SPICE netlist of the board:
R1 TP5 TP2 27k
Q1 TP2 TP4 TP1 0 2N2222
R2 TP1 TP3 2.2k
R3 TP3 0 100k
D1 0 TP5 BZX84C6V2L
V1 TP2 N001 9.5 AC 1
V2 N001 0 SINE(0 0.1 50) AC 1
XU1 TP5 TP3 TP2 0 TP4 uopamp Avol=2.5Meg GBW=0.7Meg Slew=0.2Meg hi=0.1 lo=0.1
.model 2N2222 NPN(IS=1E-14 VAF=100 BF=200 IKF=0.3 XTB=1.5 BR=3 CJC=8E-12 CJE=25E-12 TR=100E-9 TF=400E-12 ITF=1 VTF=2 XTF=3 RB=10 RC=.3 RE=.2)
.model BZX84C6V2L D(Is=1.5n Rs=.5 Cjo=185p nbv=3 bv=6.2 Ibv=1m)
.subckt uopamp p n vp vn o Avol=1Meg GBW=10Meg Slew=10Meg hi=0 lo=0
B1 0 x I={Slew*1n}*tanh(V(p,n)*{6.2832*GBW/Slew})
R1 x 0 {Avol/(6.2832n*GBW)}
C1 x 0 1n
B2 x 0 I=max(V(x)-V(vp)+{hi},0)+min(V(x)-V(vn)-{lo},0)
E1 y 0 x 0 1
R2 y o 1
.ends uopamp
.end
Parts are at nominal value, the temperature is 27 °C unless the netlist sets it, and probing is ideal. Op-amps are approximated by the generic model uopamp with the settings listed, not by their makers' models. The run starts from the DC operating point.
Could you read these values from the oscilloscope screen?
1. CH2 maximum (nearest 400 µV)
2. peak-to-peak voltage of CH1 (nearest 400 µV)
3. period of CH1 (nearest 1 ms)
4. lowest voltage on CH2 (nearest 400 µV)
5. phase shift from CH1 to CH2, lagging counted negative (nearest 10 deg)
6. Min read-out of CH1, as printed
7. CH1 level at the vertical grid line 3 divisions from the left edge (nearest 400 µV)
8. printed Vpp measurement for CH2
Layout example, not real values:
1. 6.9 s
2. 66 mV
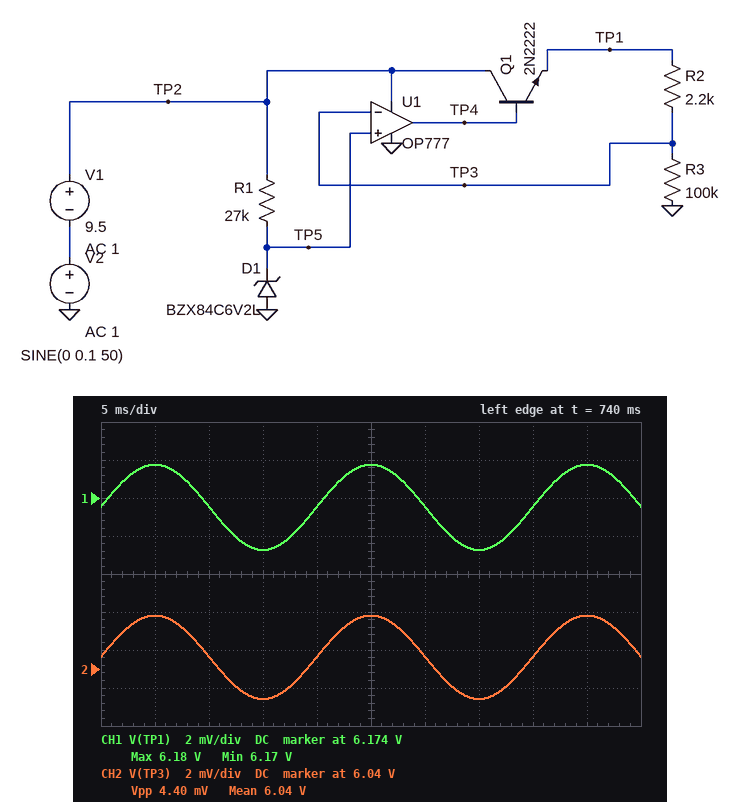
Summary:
1. 6.0428 V
2. 4.4 mV
3. 20 ms
4. 6.0384 V
5. 0 deg
6. 6.17 V
7. 6.1712 V
8. 4.40 mV
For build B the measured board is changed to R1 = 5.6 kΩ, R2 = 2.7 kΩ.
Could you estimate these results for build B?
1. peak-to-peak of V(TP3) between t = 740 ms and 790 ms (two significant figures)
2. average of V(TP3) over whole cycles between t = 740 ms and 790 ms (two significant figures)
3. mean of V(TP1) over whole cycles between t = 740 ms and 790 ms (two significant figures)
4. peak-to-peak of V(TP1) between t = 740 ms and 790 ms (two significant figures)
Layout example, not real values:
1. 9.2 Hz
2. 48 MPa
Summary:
1. 4.6 mV
2. 6.2 V
3. 6.3 V
4. 4.7 mV
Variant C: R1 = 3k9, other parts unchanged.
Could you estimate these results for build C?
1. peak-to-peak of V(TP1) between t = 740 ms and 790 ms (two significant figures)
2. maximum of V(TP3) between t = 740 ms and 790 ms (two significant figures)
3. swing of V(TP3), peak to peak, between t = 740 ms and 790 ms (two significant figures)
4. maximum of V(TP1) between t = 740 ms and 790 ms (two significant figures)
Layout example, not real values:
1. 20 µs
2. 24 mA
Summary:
1. 4.7 mV
2. 6.2 V
3. 4.6 mV
4. 6.3 V
